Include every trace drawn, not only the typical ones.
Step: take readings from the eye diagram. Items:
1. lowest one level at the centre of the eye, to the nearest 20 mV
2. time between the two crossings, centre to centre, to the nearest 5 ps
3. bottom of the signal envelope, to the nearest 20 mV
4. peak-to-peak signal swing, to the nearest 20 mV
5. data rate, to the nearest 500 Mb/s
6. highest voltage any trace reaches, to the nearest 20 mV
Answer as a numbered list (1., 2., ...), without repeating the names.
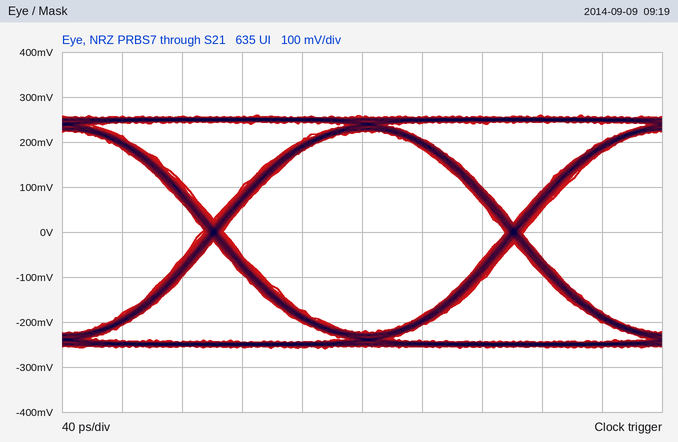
1. 220 mV
2. 200 ps
3. -260 mV
4. 520 mV
5. 5.0 Gb/s
6. 260 mV
